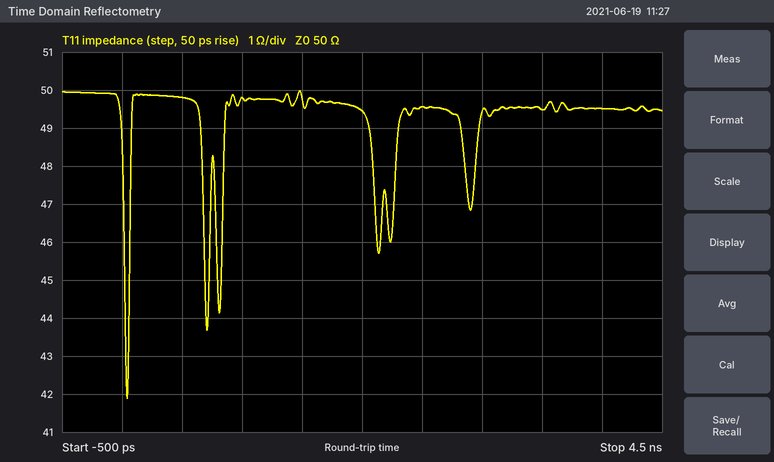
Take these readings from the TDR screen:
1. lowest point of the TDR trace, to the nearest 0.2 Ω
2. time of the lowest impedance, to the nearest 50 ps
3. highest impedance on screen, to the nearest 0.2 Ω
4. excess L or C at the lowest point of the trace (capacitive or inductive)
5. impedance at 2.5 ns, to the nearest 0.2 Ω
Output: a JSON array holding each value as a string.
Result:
["41.8 Ω", "50 ps", "50.0 Ω", "capacitive", "49.6 Ω"]
